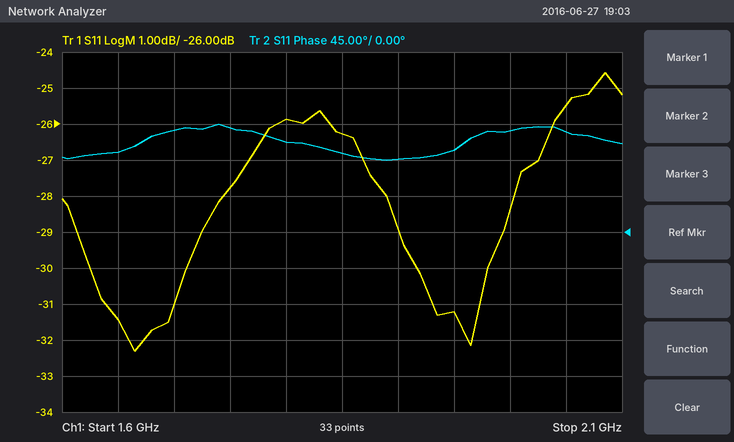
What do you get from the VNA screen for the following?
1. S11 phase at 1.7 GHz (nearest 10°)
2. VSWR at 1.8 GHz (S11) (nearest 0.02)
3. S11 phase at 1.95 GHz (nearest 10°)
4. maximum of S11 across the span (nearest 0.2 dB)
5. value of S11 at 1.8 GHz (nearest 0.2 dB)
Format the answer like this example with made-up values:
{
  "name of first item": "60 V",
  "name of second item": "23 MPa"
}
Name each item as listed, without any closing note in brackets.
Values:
{
  "S11 phase at 1.7 GHz": "130°",
  "VSWR at 1.8 GHz (S11)": "1.10",
  "S11 phase at 1.95 GHz": "100°",
  "maximum of S11 across the span": "-24.6 dB",
  "value of S11 at 1.8 GHz": "-25.8 dB"
}
